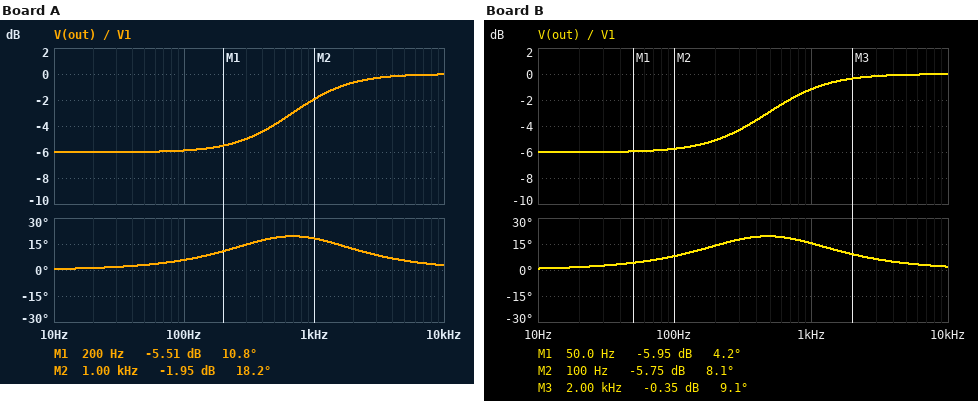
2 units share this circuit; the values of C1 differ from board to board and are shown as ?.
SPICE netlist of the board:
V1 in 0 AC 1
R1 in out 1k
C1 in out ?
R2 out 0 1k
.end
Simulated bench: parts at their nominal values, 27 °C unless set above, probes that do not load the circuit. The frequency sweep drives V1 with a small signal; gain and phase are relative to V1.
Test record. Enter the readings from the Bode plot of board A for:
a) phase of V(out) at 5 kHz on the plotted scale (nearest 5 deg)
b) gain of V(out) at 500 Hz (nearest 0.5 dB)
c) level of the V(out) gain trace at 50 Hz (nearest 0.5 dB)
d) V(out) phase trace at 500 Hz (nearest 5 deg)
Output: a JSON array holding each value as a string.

["5 deg", "-4.0 dB", "-6.0 dB", "20 deg"]
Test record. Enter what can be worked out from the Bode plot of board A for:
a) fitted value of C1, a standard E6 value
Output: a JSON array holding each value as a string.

["330 nF"]
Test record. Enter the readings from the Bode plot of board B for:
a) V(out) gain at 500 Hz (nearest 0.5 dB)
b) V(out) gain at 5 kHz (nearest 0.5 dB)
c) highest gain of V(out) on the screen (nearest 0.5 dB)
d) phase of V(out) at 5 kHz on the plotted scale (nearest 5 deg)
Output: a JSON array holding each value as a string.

["-3.0 dB", "0 dB", "0 dB", "5 deg"]
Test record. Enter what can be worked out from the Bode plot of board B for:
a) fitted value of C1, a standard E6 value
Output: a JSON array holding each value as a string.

["470 nF"]
